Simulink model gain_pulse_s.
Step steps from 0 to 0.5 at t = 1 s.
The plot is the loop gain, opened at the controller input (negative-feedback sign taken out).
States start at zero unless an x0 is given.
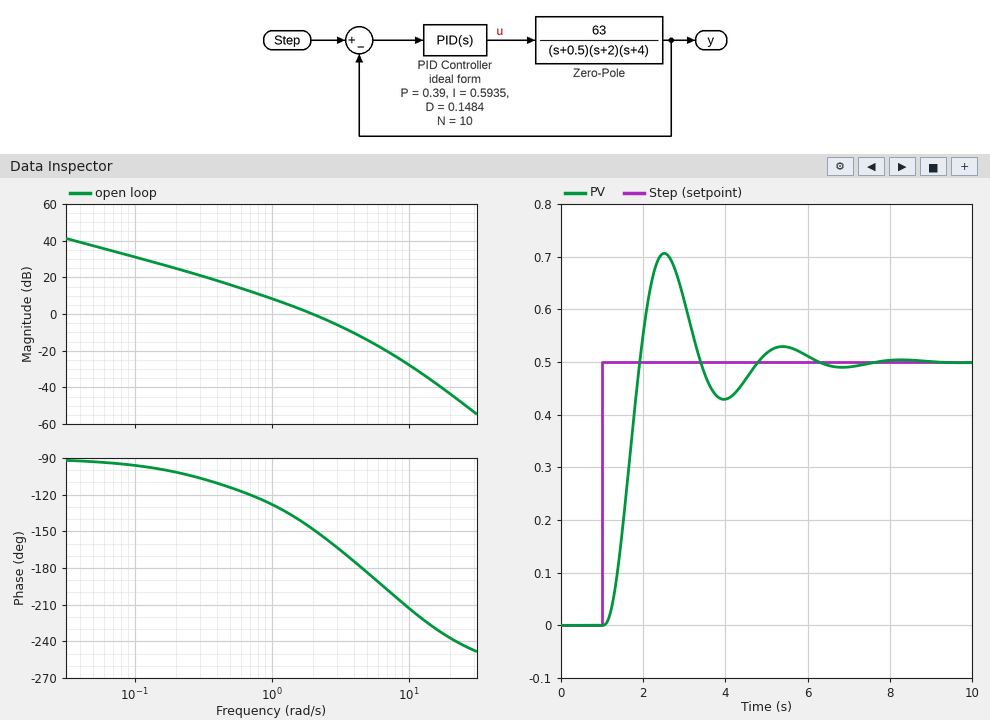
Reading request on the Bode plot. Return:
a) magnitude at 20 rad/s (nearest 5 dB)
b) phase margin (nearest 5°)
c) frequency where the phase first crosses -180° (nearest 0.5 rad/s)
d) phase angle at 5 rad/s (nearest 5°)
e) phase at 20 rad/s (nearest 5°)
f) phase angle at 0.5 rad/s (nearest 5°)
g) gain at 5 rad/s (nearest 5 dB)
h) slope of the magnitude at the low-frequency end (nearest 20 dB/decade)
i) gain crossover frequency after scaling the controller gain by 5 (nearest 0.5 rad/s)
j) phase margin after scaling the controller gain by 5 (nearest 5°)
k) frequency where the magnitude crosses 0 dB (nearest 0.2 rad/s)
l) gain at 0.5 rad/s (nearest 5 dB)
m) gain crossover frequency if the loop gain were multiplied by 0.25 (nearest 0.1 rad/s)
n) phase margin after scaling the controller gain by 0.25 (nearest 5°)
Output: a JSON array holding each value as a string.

["-45 dB", "30°", "4.5 rad/s", "-185°", "-235°", "-115°", "-15 dB", "-20 dB/decade", "5.0 rad/s", "-5°", "2.0 rad/s", "15 dB", "0.7 rad/s", "60°"]
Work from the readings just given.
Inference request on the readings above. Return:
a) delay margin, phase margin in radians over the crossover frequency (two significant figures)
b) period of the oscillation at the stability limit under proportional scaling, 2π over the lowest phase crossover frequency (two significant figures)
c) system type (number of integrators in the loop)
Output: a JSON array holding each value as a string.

["0.26 s", "1.4 s", "1"]
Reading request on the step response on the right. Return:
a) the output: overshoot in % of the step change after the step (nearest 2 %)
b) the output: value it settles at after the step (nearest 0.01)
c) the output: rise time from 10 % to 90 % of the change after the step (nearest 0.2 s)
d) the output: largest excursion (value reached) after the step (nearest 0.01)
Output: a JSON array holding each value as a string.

["42 %", "0.50", "0.6 s", "0.71"]
